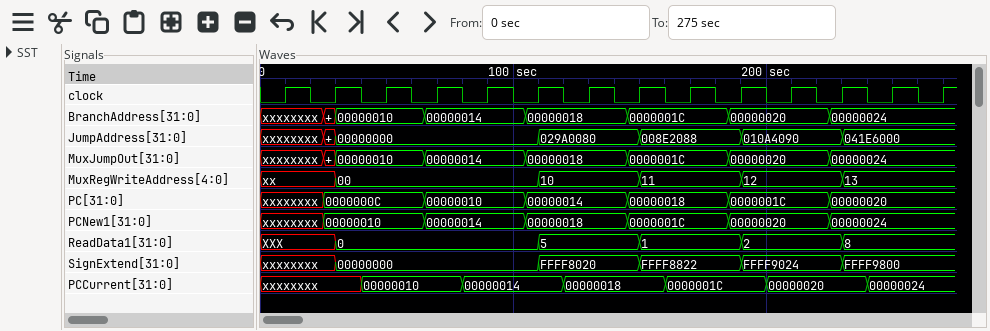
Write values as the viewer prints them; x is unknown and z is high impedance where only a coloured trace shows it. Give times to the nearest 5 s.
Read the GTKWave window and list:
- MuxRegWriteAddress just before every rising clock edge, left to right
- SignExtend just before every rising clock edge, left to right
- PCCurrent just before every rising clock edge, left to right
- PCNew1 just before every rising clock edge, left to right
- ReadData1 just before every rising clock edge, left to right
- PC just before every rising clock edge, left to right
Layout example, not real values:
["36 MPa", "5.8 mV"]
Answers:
["xx, xx, 00, 00, 00, 00, 10, 10, 11, 11, 12, 12, 13, 13", "xxxxxxxx, xxxxxxxx, 00000000, 00000000, 00000000, 00000000, FFFF8020, FFFF8020, FFFF8822, FFFF8822, FFFF9024, FFFF9024, FFFF9800, FFFF9800", "xxxxxxxx, xxxxxxxx, 00000010, 00000010, 00000014, 00000014, 00000018, 00000018, 0000001C, 0000001C, 00000020, 00000020, 00000024, 00000024", "xxxxxxxx, 00000010, 00000010, 00000014, 00000014, 00000018, 00000018, 0000001C, 0000001C, 00000020, 00000020, 00000024, 00000024, 00000024", "XXX, XXX, 0, 0, 0, 0, 5, 5, 1, 1, 2, 2, 8, 8", "xxxxxxxx, 0000000C, 0000000C, 00000010, 00000010, 00000014, 00000014, 00000018, 00000018, 0000001C, 0000001C, 00000020, 00000020, 00000020"]
